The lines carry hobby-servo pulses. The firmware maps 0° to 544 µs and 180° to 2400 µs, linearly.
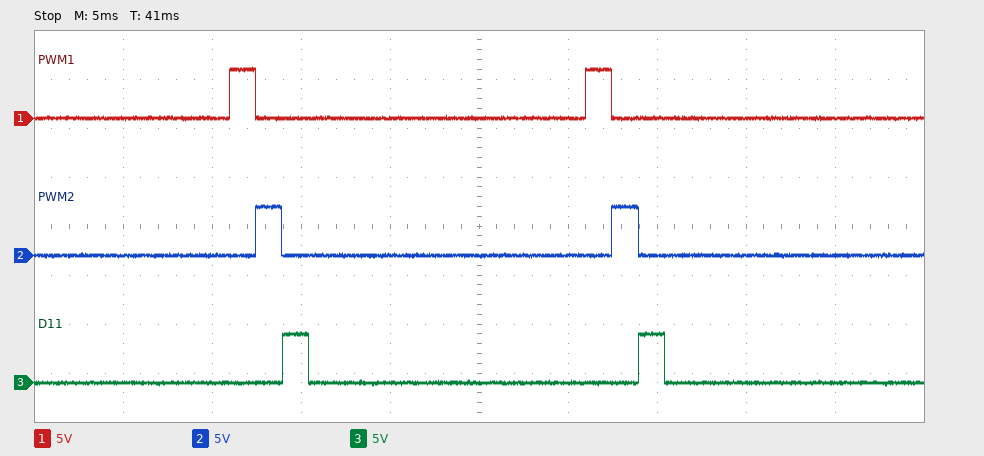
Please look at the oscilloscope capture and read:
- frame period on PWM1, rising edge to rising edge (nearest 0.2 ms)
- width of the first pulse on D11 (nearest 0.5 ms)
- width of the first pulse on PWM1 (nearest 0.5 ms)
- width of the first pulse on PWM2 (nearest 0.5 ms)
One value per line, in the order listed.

20.0 ms
1.5 ms
1.5 ms
1.5 ms
